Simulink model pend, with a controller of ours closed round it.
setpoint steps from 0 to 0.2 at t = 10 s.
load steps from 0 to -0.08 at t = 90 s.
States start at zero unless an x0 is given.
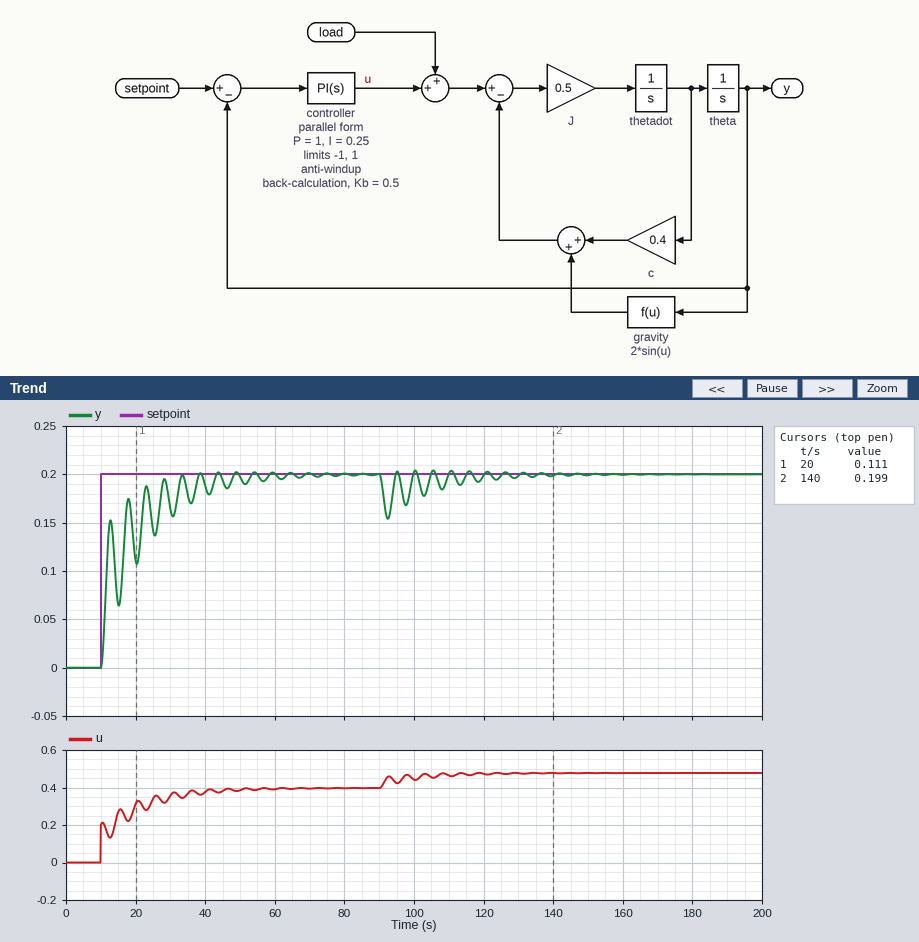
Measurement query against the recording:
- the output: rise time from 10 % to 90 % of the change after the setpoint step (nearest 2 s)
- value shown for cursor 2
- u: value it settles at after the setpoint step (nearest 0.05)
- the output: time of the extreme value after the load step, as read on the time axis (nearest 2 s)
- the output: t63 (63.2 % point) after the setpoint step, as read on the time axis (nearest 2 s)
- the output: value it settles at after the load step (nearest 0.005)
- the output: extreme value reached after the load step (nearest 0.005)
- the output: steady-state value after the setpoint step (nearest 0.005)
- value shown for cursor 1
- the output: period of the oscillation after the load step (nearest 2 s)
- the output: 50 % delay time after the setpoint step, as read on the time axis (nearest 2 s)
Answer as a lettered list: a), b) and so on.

a) 12 s
b) 0.199
c) 0.40
d) 92 s
e) 12 s
f) 0.200
g) 0.155
h) 0.200
i) 0.111
j) 6 s
k) 12 s
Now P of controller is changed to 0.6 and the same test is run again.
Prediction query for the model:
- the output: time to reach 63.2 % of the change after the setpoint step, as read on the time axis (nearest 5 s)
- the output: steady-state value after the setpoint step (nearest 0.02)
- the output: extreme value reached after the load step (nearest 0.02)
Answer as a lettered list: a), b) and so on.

a) 15 s
b) 0.20
c) 0.14
